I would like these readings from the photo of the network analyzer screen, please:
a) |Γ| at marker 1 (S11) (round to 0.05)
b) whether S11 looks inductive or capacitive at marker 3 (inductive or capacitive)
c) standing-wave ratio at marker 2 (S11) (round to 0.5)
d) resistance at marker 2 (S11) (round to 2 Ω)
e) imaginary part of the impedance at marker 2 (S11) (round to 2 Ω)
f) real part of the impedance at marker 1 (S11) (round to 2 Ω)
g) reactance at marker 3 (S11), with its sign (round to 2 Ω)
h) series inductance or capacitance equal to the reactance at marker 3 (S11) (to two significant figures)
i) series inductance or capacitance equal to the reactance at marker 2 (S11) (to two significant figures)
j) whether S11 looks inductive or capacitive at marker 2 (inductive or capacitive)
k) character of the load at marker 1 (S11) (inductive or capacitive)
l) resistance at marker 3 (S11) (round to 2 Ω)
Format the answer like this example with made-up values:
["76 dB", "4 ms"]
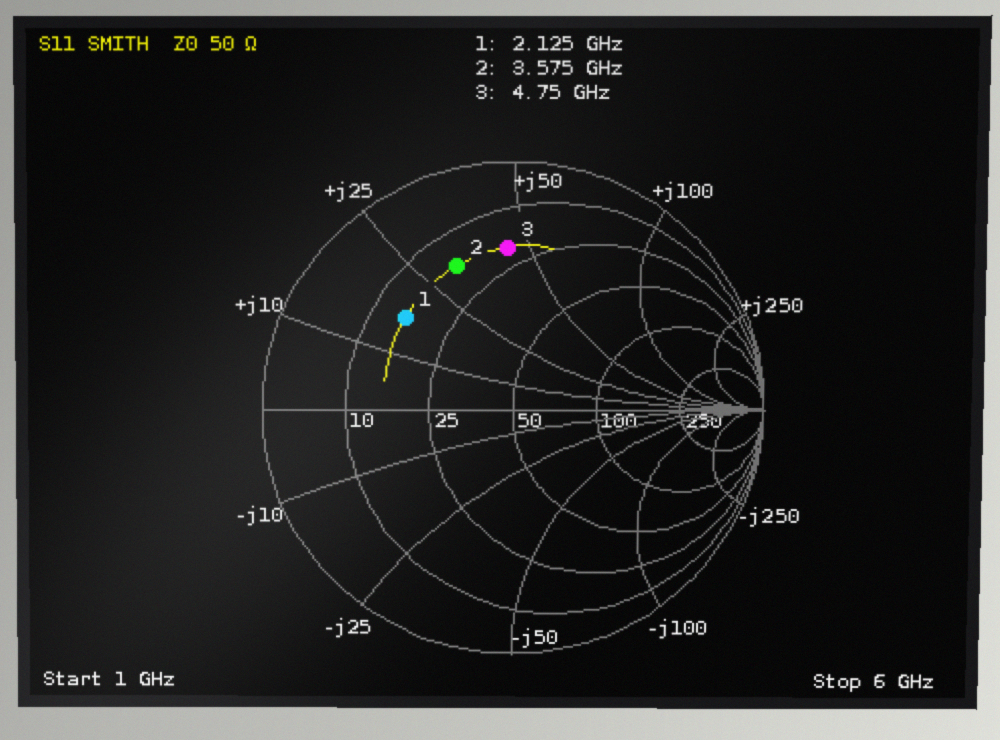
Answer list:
["0.55", "inductive", "4.5", "16 Ω", "+32 Ω", "16 Ω", "+44 Ω", "1.5 nH", "1.4 nH", "inductive", "inductive", "20 Ω"]
